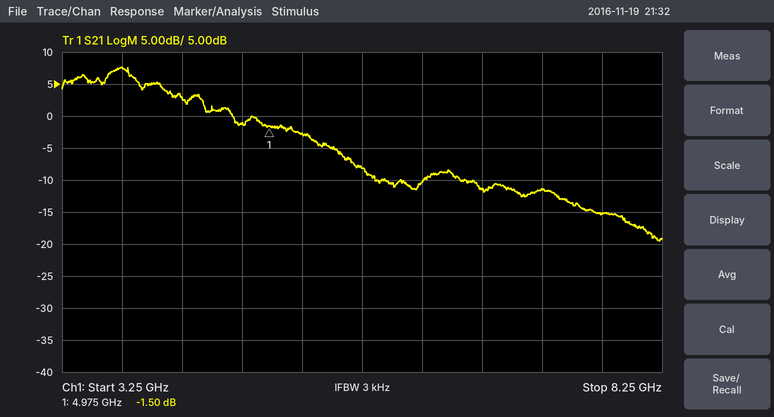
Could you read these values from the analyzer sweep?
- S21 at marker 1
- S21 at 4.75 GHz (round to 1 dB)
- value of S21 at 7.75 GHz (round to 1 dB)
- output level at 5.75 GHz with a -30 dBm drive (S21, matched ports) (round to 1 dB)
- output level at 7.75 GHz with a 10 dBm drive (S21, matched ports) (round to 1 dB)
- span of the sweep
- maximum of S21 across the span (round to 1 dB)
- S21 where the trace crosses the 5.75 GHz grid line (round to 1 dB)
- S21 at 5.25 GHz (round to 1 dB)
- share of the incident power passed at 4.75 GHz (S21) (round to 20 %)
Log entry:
-1.50 dB
-1 dB
-15 dB
-38 dBm
-5 dBm
5 GHz
8 dB
-8 dB
-3 dB
80 %
